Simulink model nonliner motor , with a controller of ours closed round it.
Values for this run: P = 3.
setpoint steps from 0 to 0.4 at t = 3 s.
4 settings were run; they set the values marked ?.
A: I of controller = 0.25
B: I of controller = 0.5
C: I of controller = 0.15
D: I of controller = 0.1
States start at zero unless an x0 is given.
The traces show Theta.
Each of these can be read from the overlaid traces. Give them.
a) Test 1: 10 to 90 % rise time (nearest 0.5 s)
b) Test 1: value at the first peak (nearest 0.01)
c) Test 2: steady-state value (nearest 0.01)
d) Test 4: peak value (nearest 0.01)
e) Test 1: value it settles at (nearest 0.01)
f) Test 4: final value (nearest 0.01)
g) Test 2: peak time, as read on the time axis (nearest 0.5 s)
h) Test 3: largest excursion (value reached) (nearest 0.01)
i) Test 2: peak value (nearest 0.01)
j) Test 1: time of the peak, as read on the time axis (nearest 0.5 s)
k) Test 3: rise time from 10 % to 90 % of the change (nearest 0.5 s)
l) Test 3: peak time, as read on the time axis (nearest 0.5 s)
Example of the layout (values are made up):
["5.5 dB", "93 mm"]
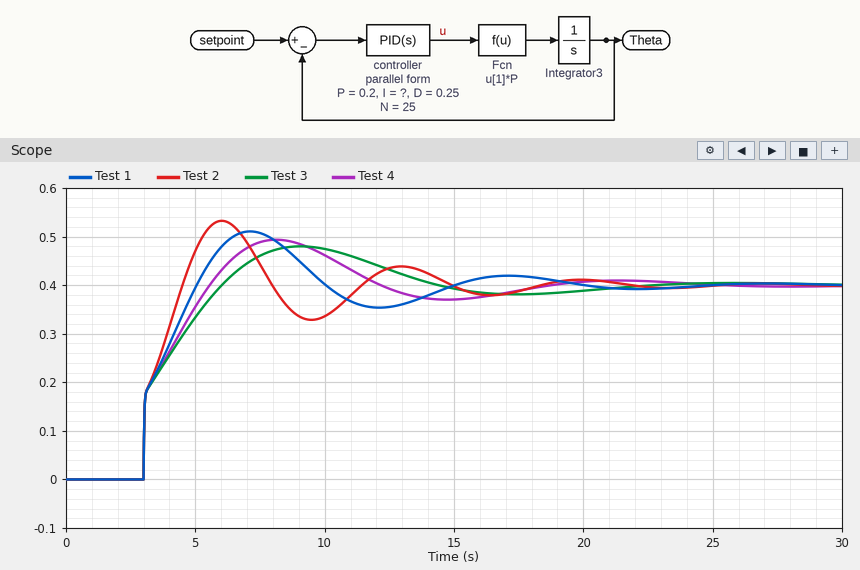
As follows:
["1.5 s", "0.51", "0.40", "0.49", "0.40", "0.40", "6.0 s", "0.48", "0.53", "7.0 s", "2.5 s", "9.0 s"]
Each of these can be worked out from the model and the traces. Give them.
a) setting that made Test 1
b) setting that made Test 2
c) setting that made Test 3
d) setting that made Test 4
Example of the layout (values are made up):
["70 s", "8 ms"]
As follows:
["A", "B", "D", "C"]
